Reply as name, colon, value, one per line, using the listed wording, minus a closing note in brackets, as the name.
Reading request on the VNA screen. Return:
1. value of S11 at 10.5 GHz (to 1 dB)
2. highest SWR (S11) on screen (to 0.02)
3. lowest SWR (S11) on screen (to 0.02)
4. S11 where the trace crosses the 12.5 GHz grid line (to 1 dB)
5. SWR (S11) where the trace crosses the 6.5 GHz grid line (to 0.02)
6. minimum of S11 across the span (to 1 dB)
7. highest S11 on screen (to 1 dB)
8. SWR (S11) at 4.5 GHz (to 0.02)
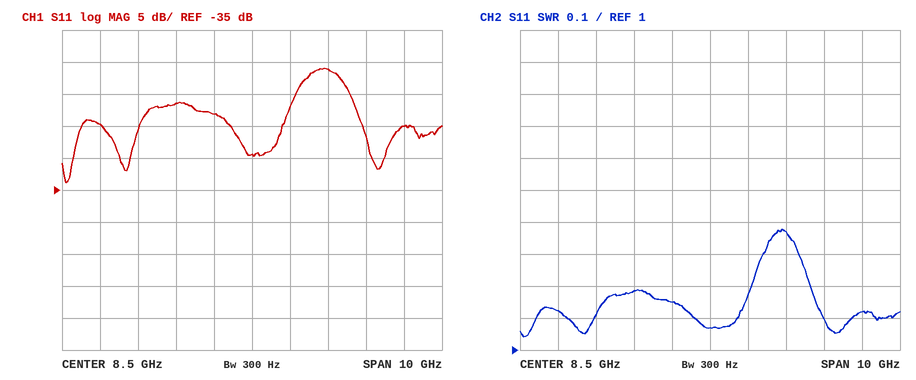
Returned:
value of S11 at 10.5 GHz: -16 dB
highest SWR (S11) on screen: 1.38
lowest SWR (S11) on screen: 1.04
S11 where the trace crosses the 12.5 GHz grid line: -25 dB
SWR (S11) where the trace crosses the 6.5 GHz grid line: 1.18
minimum of S11 across the span: -34 dB
highest S11 on screen: -16 dB
SWR (S11) at 4.5 GHz: 1.12
